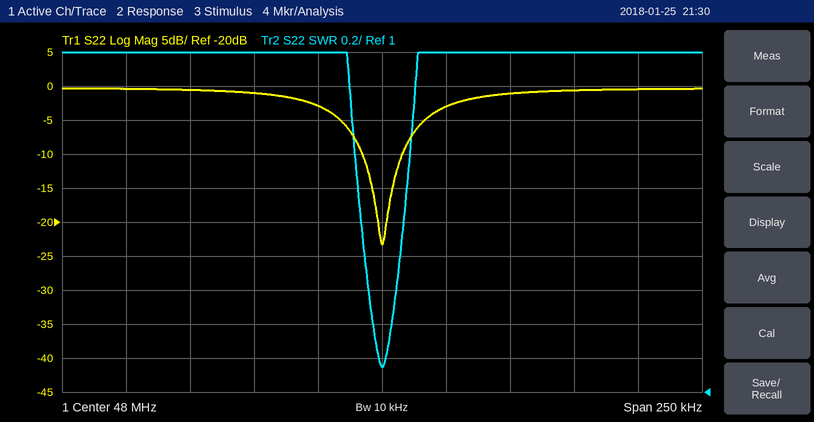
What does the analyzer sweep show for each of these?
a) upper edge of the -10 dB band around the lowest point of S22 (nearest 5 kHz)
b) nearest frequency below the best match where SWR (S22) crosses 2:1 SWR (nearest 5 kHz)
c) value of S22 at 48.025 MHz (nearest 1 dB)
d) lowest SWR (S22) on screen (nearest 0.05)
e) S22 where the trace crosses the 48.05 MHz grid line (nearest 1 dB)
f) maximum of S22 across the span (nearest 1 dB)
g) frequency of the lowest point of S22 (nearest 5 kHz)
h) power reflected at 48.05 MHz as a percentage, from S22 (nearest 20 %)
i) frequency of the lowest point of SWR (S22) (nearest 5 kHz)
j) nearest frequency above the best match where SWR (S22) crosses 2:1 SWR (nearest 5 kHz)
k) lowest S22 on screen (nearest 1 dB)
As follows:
48.010 MHz
47.990 MHz
-3 dB
1.15
-1 dB
0 dB
48.000 MHz
80 %
48.000 MHz
48.010 MHz
-23 dB
